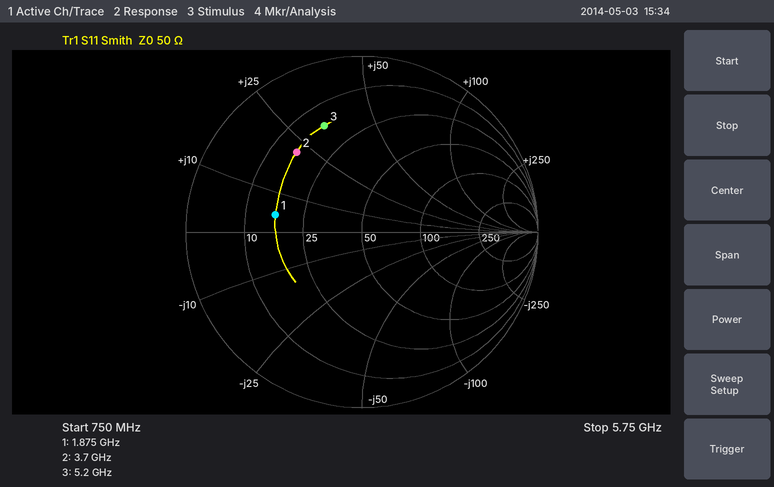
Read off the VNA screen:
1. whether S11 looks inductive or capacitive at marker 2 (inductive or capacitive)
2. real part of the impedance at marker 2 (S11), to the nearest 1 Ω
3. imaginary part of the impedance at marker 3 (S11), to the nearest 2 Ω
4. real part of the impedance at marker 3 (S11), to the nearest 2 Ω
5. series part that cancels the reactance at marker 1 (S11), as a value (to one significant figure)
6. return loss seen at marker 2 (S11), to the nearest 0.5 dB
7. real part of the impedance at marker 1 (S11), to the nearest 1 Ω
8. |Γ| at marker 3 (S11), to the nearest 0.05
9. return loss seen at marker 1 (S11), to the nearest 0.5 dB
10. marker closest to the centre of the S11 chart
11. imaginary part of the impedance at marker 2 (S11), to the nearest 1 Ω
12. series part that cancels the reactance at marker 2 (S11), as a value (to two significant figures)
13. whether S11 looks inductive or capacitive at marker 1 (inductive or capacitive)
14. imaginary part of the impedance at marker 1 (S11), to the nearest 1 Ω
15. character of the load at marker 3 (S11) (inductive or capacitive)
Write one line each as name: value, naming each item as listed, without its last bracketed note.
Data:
whether S11 looks inductive or capacitive at marker 2: inductive
real part of the impedance at marker 2 (S11), to the nearest 1 Ω: 16 Ω
imaginary part of the impedance at marker 3 (S11), to the nearest 2 Ω: +32 Ω
real part of the impedance at marker 3 (S11), to the nearest 2 Ω: 16 Ω
series part that cancels the reactance at marker 1 (S11), as a value: 20 pF
return loss seen at marker 2 (S11), to the nearest 0.5 dB: 4.5 dB
real part of the impedance at marker 1 (S11), to the nearest 1 Ω: 17 Ω
|Γ| at marker 3 (S11), to the nearest 0.05: 0.65
return loss seen at marker 1 (S11), to the nearest 0.5 dB: 6.0 dB
marker closest to the centre of the S11 chart: marker 1
imaginary part of the impedance at marker 2 (S11), to the nearest 1 Ω: +22 Ω
series part that cancels the reactance at marker 2 (S11), as a value: 2.0 pF
whether S11 looks inductive or capacitive at marker 1: inductive
imaginary part of the impedance at marker 1 (S11), to the nearest 1 Ω: +4 Ω
character of the load at marker 3 (S11): inductive
